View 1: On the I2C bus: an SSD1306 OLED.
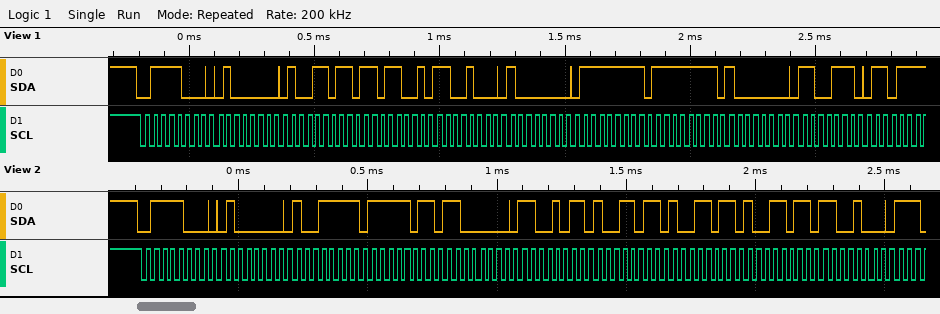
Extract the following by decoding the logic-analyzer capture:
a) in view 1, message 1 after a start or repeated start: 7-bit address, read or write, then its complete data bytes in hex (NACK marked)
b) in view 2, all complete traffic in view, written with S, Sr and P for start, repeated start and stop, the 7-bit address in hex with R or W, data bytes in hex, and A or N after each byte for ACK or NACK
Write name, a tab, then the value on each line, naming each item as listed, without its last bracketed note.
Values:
in view 1, message 1 after a start or repeated start: 7-bit address, read or write, then its complete data bytes in hex	0x3C write: 40 9B D9 C8 80 FF FF 80 CE
in view 2, all complete traffic in view, written with S, Sr and P for start, repeated start and stop, the 7-bit address in hex with R or W, data bytes in hex, and A or N after each byte for ACK or NACK	S 3CW A 40 A 9F A FB A C0 A CB A 9B A 9B A 9B A C8 A
